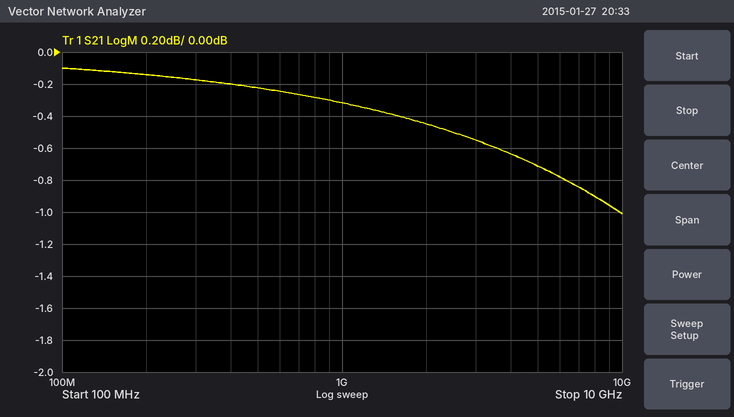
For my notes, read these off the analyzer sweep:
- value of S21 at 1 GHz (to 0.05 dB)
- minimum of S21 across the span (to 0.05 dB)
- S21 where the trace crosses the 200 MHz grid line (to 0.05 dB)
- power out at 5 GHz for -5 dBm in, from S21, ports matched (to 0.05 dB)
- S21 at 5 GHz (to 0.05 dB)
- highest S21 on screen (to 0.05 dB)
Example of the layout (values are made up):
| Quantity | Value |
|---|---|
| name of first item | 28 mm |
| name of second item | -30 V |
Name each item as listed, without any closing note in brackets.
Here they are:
| Quantity | Value |
|---|---|
| value of S21 at 1 GHz | -0.30 dB |
| minimum of S21 across the span | -1.00 dB |
| S21 where the trace crosses the 200 MHz grid line | -0.15 dB |
| power out at 5 GHz for -5 dBm in, from S21, ports matched | -5.70 dBm |
| S21 at 5 GHz | -0.70 dB |
| highest S21 on screen | -0.10 dB |
